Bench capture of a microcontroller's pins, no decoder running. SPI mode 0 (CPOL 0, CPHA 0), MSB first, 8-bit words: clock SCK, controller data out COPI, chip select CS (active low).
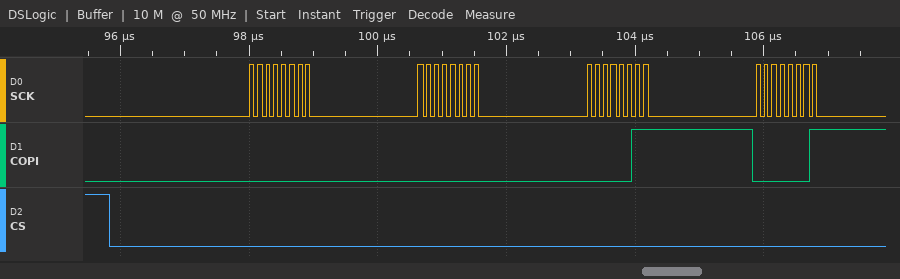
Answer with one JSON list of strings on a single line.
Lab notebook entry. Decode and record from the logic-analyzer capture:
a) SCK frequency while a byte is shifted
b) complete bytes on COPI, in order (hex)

["8 MHz", "0x00 0x00 0x03 0x01"]
